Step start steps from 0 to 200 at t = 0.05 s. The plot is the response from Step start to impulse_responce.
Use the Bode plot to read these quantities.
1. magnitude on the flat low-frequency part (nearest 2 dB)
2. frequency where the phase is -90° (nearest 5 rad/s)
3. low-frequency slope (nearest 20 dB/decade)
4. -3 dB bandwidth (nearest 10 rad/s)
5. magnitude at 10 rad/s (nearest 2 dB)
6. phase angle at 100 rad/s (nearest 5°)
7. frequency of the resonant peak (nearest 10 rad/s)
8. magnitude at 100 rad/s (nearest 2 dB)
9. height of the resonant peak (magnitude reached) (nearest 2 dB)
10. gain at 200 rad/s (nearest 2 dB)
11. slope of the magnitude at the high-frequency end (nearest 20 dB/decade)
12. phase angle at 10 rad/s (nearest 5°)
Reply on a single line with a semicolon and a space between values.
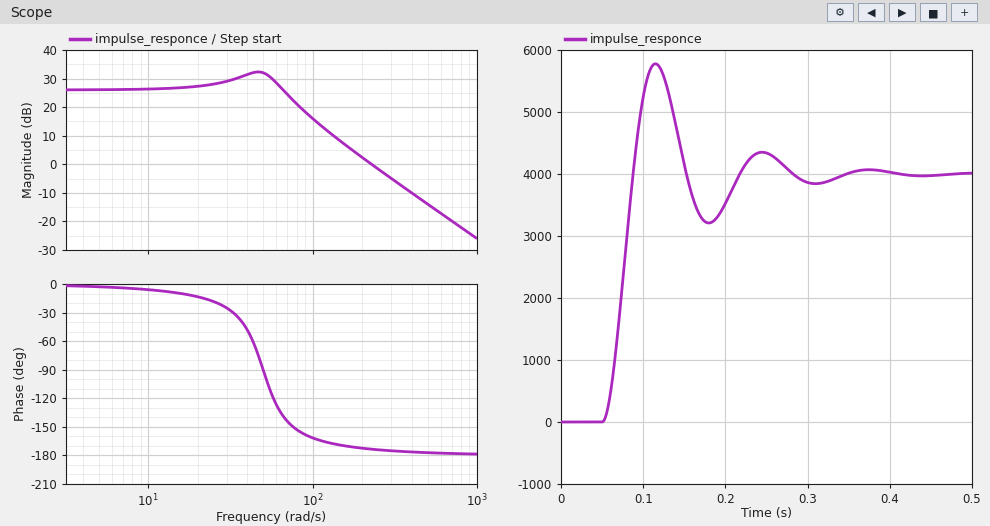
26 dB; 50 rad/s; 0 dB/decade; 70 rad/s; 26 dB; -160°; 50 rad/s; 16 dB; 32 dB; 2 dB; -40 dB/decade; -5°
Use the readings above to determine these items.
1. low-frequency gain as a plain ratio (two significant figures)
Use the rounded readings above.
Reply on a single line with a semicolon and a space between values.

20
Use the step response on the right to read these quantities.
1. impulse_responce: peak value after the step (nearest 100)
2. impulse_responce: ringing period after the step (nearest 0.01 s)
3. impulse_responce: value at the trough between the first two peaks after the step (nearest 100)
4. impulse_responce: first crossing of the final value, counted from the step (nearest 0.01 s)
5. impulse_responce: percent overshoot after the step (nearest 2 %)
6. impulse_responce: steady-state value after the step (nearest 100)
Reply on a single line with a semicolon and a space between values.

5800; 0.13 s; 3200; 0.04 s; 44 %; 4000
